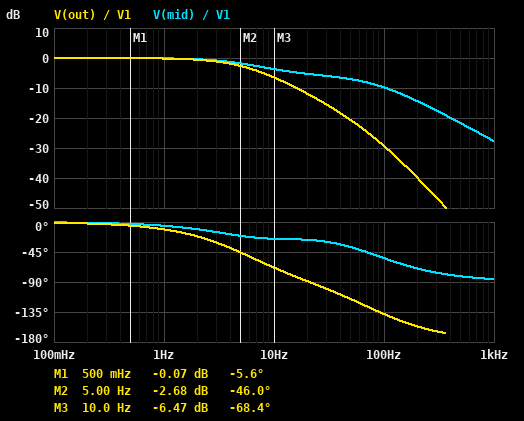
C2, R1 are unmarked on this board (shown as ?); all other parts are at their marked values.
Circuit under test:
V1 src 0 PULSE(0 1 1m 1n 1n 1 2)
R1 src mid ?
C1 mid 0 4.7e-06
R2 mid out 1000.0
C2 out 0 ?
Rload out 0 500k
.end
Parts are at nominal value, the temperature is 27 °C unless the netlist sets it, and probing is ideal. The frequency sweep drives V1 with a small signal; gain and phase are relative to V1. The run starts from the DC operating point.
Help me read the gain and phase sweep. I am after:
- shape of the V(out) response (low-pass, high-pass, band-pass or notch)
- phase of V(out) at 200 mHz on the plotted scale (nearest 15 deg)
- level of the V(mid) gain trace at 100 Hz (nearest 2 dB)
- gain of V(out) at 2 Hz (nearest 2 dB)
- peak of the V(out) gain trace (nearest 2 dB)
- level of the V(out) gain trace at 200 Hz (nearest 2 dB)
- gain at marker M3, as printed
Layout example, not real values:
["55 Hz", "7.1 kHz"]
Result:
["low-pass", "0 deg", "-10 dB", "0 dB", "0 dB", "-40 dB", "-6.47 dB"]
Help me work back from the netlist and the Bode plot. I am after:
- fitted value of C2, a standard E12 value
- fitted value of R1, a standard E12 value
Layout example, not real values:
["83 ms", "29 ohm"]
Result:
["15 µF", "820 Ω"]
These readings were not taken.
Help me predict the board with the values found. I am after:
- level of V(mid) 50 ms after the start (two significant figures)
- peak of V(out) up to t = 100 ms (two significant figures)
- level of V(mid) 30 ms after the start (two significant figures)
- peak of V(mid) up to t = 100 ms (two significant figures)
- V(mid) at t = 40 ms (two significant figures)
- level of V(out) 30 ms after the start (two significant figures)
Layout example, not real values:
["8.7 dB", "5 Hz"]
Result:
["900 mV", "960 mV", "810 mV", "980 mV", "860 mV", "600 mV"]
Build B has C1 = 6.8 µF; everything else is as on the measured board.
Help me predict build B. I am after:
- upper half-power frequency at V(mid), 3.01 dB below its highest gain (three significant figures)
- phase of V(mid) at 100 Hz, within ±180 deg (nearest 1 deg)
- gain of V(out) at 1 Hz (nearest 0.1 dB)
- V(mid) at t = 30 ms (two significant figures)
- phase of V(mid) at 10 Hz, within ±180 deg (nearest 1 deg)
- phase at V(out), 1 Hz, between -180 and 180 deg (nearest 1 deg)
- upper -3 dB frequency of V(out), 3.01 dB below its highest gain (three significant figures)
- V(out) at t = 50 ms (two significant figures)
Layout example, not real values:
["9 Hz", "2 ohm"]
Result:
["7.31 Hz", "-63 deg", "-0.2 dB", "790 mV", "-29 deg", "-12 deg", "5.26 Hz", "780 mV"]
